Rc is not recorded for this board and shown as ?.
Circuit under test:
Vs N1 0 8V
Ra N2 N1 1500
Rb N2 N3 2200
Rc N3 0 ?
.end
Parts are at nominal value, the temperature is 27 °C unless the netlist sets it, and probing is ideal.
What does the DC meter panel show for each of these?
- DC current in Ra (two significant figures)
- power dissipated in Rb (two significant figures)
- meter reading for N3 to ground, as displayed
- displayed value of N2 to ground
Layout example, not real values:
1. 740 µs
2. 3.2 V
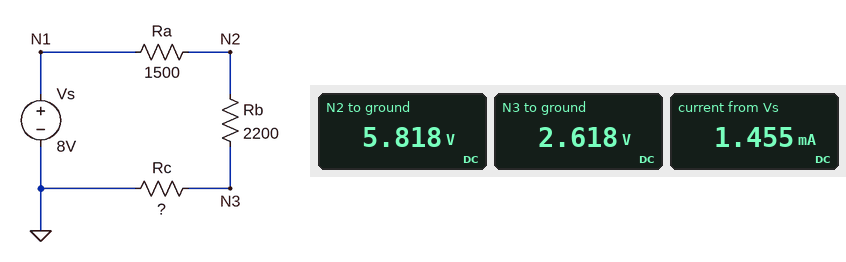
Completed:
1. 1.5 mA
2. 4.7 mW
3. 2.618 V
4. 5.818 V
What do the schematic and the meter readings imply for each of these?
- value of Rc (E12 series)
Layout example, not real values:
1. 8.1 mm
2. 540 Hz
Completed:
1. 1.8 kΩ
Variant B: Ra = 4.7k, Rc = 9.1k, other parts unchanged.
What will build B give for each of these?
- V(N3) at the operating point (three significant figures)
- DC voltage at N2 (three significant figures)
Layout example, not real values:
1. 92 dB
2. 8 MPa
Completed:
1. 4.55 V
2. 5.65 V
